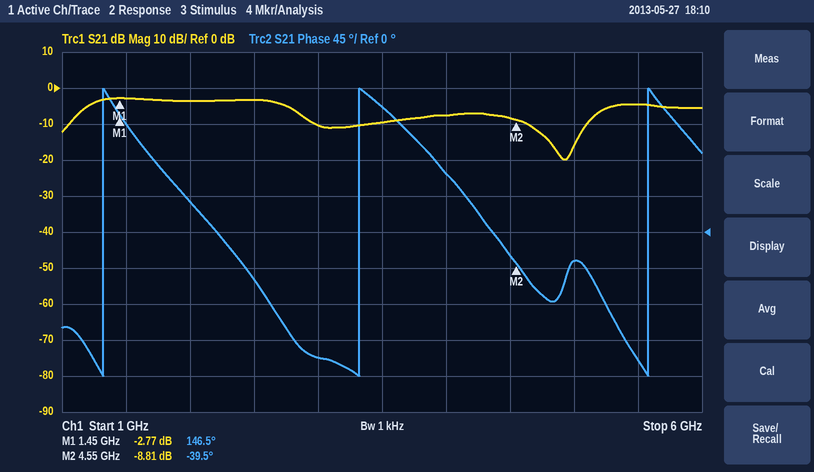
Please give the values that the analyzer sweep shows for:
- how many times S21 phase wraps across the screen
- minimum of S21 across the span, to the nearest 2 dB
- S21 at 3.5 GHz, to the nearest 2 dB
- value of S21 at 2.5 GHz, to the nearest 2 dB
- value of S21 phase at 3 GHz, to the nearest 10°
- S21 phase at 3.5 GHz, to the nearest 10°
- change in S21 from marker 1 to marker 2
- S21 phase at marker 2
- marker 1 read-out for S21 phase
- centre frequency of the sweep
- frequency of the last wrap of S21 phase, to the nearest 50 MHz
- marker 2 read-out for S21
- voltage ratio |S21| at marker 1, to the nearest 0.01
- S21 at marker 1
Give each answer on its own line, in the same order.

3
-20 dB
-10 dB
-4 dB
-160°
160°
-6.04 dB
-39.5°
146.5°
3.5 GHz
5.60 GHz
-8.81 dB
0.73
-2.77 dB
